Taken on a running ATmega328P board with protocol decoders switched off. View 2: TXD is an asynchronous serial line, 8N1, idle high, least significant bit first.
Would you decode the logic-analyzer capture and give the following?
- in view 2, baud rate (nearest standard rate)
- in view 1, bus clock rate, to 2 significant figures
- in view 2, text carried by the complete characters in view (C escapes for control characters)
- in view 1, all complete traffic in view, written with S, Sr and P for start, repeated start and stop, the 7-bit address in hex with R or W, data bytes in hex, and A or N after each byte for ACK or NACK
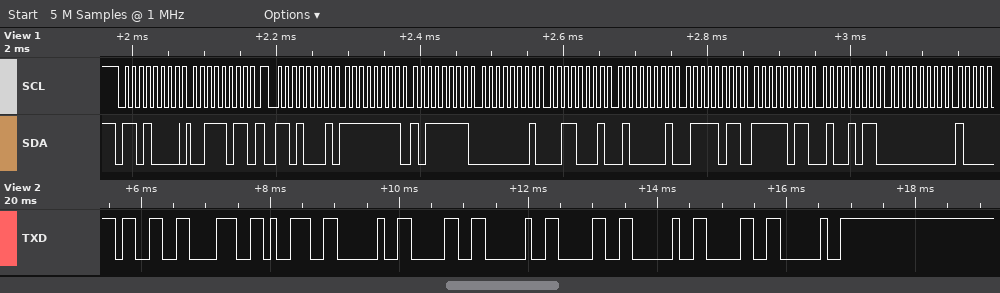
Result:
9600 baud
100 kHz
"389 0 0 0 "
S 68W A 3B A Sr 68R A FF A BF A 01 A 31 A 41 A 7B A FB A 4B A 00 A
